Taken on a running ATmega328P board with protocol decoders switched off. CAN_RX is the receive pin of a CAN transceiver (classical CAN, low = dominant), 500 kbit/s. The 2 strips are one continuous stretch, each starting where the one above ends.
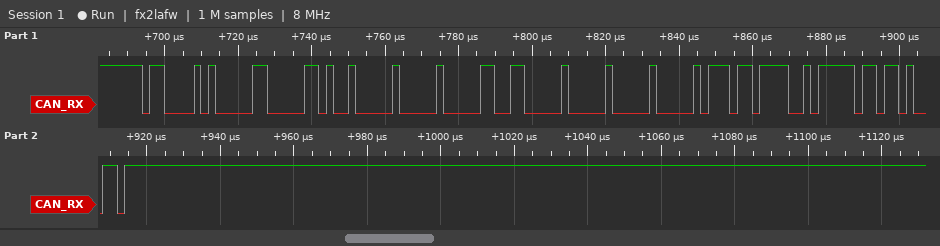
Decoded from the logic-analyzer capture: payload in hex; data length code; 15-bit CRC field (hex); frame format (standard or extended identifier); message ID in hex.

29 00 01 30 00 00 76 F2
8
0x7F69
standard
0x614
